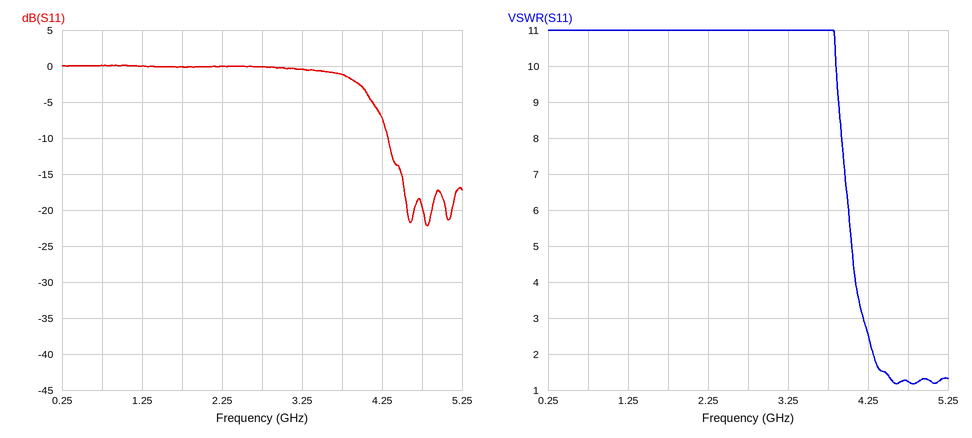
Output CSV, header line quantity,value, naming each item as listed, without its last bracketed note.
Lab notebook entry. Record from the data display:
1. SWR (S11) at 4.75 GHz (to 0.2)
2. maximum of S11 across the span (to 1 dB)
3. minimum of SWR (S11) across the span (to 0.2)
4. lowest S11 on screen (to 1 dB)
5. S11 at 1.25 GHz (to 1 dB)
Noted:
quantity,value
SWR (S11) at 4.75 GHz,1.2
maximum of S11 across the span,0 dB
minimum of SWR (S11) across the span,1.2
lowest S11 on screen,-22 dB
S11 at 1.25 GHz,0 dB
